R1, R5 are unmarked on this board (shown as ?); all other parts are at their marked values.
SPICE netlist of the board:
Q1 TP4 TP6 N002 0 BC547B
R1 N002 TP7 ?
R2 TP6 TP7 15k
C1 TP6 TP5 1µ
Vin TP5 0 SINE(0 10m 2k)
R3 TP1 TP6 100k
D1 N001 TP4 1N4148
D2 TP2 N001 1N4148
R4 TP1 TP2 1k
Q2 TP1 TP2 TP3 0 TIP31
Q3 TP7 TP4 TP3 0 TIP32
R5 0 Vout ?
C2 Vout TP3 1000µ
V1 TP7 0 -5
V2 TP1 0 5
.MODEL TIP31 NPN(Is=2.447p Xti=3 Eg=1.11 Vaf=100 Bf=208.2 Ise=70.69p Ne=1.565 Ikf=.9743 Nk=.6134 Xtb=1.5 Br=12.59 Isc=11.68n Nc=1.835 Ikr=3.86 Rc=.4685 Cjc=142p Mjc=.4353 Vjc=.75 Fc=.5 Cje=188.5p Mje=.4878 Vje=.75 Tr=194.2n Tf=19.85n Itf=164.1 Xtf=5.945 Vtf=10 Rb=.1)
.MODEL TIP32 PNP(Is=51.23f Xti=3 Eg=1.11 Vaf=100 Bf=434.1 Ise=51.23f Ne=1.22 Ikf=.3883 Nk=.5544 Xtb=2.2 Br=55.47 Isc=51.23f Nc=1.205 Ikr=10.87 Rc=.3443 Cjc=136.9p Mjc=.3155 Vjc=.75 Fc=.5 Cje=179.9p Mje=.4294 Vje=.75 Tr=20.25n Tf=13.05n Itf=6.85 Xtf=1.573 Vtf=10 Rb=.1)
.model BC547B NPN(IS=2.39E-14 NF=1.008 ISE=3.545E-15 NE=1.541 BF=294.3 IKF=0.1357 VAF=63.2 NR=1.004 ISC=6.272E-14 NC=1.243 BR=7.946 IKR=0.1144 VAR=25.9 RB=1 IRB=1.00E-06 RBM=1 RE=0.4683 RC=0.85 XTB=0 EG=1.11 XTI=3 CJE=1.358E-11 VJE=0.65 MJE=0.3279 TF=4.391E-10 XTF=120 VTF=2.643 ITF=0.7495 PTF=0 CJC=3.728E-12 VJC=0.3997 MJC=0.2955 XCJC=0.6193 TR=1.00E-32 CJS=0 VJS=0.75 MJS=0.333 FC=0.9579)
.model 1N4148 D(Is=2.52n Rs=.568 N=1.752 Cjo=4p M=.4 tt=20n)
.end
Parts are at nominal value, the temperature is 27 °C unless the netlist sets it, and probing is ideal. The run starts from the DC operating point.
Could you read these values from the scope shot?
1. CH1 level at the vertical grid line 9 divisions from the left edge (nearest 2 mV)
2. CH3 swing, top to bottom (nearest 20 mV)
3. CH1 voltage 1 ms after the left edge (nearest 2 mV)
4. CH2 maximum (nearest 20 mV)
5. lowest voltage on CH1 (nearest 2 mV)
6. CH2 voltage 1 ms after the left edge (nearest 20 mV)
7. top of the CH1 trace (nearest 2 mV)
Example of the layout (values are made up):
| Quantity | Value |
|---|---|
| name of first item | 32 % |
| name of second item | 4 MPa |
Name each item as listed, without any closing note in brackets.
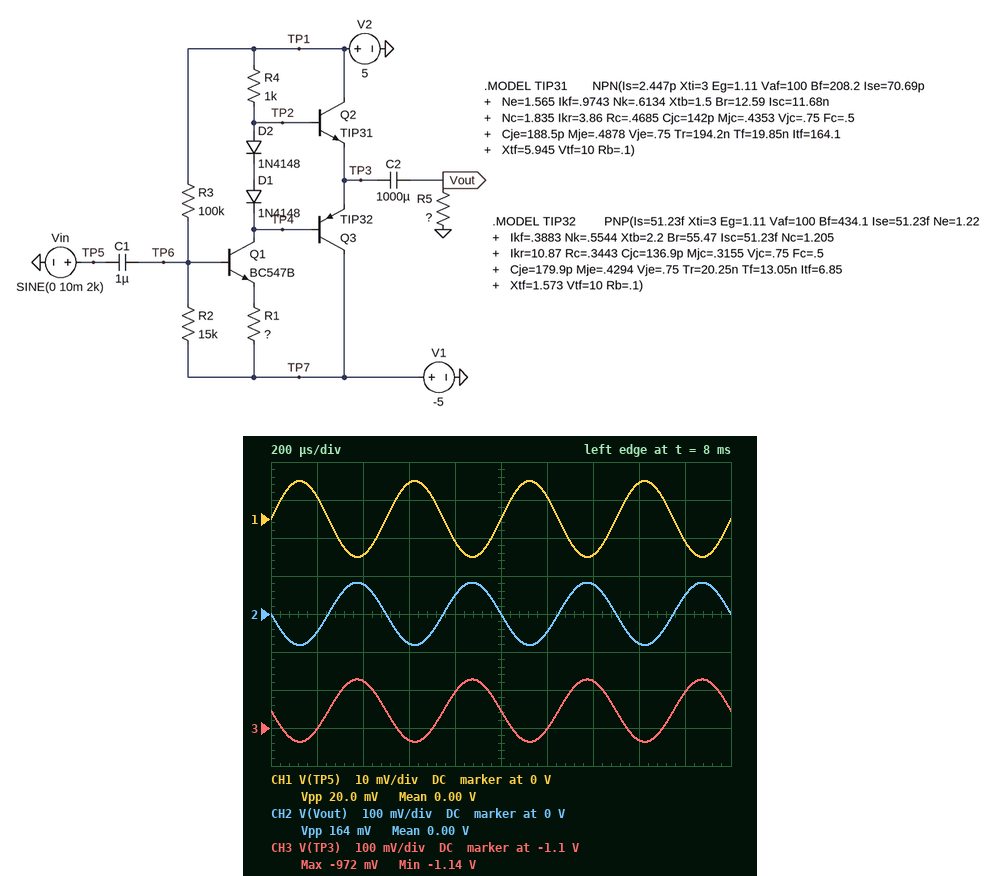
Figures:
| Quantity | Value |
|---|---|
| CH1 level at the vertical grid line 9 divisions from the left edge | -6 mV |
| CH3 swing, top to bottom | 160 mV |
| CH1 voltage 1 ms after the left edge | 0 V |
| CH2 maximum | 80 mV |
| lowest voltage on CH1 | -10 mV |
| CH2 voltage 1 ms after the left edge | 0 V |
| top of the CH1 trace | 10 mV |
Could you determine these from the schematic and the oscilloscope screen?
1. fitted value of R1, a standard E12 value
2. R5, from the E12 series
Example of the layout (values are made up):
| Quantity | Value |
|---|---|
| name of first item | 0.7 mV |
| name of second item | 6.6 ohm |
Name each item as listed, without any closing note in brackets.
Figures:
| Quantity | Value |
|---|---|
| fitted value of R1, a standard E12 value | 68 Ω |
| R5, from the E12 series | 15 Ω |
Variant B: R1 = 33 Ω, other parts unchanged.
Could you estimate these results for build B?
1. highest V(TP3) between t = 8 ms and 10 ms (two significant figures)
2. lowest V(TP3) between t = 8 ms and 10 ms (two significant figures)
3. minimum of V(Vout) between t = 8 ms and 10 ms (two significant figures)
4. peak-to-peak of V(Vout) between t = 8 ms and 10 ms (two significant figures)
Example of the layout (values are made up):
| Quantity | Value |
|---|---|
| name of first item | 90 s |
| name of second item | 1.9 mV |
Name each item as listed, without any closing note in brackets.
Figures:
| Quantity | Value |
|---|---|
| highest V(TP3) between t = 8 ms and 10 ms | -2.9 V |
| lowest V(TP3) between t = 8 ms and 10 ms | -3.2 V |
| minimum of V(Vout) between t = 8 ms and 10 ms | -160 mV |
| peak-to-peak of V(Vout) between t = 8 ms and 10 ms | 320 mV |
